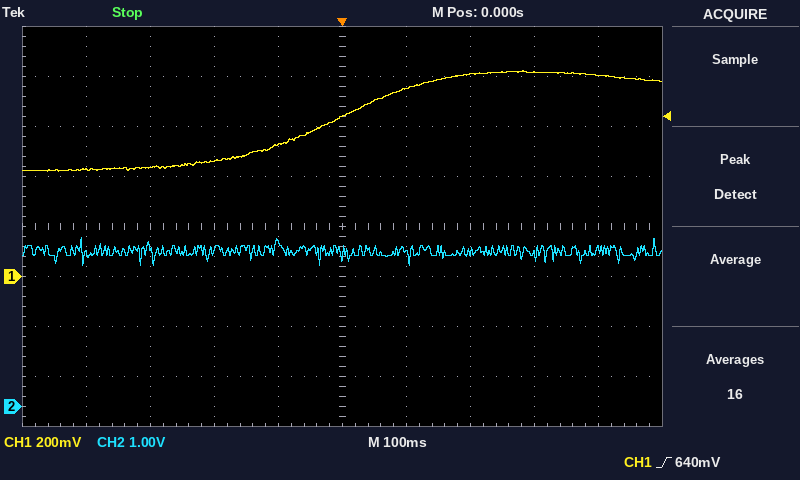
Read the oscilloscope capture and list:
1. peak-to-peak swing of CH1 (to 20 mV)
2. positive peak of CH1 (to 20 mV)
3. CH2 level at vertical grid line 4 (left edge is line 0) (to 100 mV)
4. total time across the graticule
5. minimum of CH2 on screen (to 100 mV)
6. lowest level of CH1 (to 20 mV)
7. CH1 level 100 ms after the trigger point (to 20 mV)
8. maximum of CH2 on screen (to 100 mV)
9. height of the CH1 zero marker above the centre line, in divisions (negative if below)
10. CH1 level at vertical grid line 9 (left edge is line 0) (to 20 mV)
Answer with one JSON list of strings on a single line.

["400 mV", "820 mV", "3.3 V", "1 s", "2.8 V", "420 mV", "760 mV", "3.4 V", "-1.0 div", "800 mV"]
